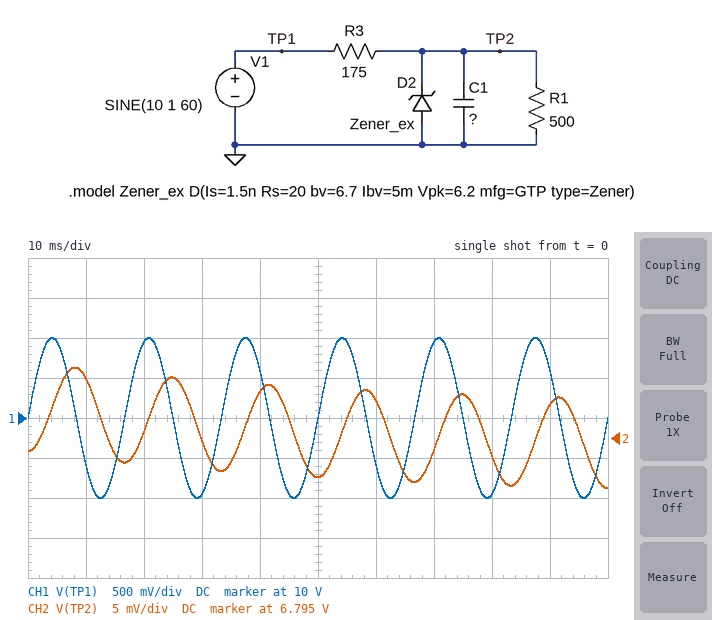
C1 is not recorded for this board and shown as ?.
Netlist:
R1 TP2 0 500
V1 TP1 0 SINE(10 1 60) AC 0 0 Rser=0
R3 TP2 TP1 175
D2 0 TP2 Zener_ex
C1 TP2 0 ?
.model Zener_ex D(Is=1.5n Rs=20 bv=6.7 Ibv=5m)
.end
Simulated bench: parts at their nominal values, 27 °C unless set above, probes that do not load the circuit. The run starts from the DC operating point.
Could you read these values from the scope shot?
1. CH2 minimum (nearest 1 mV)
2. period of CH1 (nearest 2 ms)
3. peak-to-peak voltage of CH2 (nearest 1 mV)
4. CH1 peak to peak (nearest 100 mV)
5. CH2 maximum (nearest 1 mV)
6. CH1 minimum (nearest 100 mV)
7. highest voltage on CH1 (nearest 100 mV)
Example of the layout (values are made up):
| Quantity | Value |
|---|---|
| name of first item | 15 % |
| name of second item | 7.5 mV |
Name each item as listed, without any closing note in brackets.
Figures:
| Quantity | Value |
|---|---|
| CH2 minimum | 6.789 V |
| period of CH1 | 16 ms |
| peak-to-peak voltage of CH2 | 15 mV |
| CH1 peak to peak | 2.0 V |
| CH2 maximum | 6.804 V |
| CH1 minimum | 9.0 V |
| highest voltage on CH1 | 11.0 V |
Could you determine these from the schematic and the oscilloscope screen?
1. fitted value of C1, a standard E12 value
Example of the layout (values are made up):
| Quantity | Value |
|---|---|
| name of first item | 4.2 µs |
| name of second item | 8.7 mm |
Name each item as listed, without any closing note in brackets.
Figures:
| Quantity | Value |
|---|---|
| fitted value of C1, a standard E12 value | 2.7 mF |
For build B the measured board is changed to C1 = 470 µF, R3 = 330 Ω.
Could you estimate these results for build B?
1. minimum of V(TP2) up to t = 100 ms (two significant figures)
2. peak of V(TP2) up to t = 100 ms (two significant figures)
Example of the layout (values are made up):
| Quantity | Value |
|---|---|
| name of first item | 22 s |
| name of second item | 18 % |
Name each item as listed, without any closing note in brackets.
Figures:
| Quantity | Value |
|---|---|
| minimum of V(TP2) up to t = 100 ms | 6.0 V |
| peak of V(TP2) up to t = 100 ms | 6.1 V |
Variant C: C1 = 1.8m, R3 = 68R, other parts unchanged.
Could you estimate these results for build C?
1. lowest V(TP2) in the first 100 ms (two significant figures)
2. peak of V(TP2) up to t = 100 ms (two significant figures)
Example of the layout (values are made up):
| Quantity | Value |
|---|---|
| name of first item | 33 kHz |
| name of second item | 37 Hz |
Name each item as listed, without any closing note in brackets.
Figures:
| Quantity | Value |
|---|---|
| lowest V(TP2) in the first 100 ms | 7.2 V |
| peak of V(TP2) up to t = 100 ms | 7.3 V |
